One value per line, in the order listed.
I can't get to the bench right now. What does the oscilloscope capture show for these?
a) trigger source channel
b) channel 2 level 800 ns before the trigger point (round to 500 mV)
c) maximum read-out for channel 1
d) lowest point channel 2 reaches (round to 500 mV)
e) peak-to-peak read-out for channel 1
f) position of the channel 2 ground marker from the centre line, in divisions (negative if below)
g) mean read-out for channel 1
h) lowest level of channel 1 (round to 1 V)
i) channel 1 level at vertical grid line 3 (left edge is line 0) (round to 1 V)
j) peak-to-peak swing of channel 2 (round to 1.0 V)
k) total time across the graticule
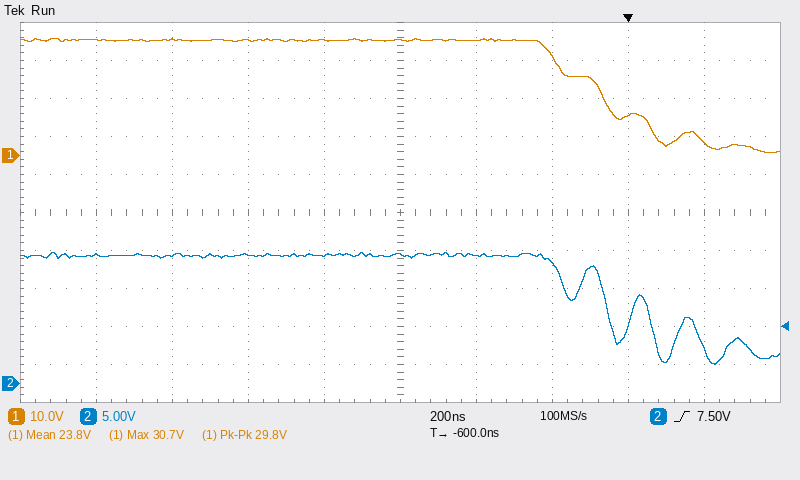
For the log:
channel 2
17.0 V
30.7 V
2.5 V
29.8 V
-4.5 div
23.8 V
1 V
30 V
15.0 V
2 µs
